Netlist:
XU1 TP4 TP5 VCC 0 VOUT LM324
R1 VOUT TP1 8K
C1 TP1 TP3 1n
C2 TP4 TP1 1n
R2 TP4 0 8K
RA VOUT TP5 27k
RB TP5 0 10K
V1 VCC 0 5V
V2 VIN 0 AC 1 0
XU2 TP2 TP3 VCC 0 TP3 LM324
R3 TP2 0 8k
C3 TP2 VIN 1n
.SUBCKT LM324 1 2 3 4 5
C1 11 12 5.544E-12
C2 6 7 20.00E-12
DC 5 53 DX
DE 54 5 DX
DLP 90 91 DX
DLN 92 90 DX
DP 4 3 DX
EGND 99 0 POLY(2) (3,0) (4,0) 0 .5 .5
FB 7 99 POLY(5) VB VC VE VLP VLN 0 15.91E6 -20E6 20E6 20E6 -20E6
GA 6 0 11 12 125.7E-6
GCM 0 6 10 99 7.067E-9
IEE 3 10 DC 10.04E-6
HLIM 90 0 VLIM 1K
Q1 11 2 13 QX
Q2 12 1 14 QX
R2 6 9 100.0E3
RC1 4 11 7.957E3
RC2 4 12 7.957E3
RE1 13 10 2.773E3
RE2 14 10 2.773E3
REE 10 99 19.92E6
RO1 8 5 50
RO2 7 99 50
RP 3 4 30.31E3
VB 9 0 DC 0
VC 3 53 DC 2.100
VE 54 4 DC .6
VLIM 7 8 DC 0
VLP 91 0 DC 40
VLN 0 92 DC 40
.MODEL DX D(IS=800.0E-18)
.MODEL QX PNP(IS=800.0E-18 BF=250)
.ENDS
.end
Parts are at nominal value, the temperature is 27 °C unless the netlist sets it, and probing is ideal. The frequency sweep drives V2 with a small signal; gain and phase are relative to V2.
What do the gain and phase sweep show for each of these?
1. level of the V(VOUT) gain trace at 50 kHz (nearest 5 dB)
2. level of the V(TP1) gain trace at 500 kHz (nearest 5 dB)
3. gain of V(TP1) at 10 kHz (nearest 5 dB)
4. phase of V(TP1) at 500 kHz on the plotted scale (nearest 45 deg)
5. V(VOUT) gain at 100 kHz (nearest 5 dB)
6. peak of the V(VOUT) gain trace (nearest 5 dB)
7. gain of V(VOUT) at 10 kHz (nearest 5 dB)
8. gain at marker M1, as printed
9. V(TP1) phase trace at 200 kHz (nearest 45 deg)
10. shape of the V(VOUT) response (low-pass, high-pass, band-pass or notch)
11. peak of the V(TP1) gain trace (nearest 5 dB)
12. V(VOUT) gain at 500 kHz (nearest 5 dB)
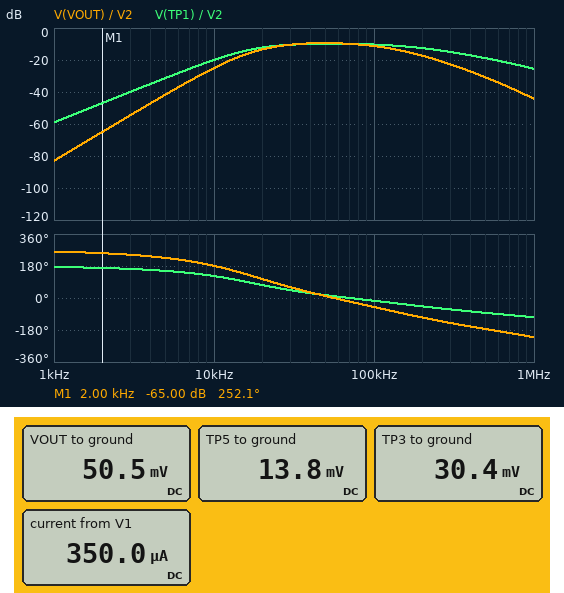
-10 dB
-20 dB
-20 dB
-90 deg
-10 dB
-10 dB
-25 dB
-65.00 dB
-45 deg
band-pass
-10 dB
-30 dB
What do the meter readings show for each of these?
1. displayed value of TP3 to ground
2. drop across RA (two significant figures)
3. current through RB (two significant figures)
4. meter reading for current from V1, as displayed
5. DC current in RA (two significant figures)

30.4 mV
37 mV
1.4 µA
350.0 µA
1.4 µA
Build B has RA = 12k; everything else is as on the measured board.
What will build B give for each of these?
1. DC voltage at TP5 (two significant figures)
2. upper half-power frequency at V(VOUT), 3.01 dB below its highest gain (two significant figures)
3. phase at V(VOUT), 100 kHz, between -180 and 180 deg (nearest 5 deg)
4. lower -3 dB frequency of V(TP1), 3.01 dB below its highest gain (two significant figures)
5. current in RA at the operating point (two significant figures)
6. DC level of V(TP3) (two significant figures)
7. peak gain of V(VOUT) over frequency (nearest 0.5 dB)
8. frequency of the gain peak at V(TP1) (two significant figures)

19 mV
130 kHz
-45 deg
23 kHz
1.9 µA
30 mV
-13.0 dB
68 kHz
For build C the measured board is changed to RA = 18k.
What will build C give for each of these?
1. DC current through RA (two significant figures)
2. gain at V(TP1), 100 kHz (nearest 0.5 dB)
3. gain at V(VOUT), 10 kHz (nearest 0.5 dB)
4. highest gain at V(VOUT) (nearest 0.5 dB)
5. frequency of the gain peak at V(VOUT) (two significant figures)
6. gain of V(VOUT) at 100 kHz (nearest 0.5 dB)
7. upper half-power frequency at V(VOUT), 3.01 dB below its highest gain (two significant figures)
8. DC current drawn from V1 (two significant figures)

1.6 µA
-10.0 dB
-27.5 dB
-11.5 dB
54 kHz
-13.0 dB
130 kHz
350 µA
